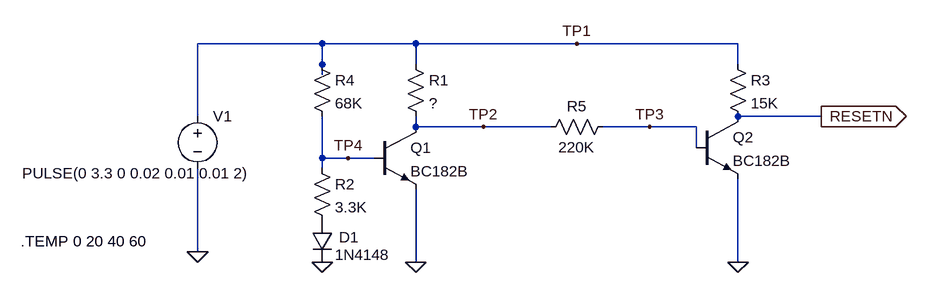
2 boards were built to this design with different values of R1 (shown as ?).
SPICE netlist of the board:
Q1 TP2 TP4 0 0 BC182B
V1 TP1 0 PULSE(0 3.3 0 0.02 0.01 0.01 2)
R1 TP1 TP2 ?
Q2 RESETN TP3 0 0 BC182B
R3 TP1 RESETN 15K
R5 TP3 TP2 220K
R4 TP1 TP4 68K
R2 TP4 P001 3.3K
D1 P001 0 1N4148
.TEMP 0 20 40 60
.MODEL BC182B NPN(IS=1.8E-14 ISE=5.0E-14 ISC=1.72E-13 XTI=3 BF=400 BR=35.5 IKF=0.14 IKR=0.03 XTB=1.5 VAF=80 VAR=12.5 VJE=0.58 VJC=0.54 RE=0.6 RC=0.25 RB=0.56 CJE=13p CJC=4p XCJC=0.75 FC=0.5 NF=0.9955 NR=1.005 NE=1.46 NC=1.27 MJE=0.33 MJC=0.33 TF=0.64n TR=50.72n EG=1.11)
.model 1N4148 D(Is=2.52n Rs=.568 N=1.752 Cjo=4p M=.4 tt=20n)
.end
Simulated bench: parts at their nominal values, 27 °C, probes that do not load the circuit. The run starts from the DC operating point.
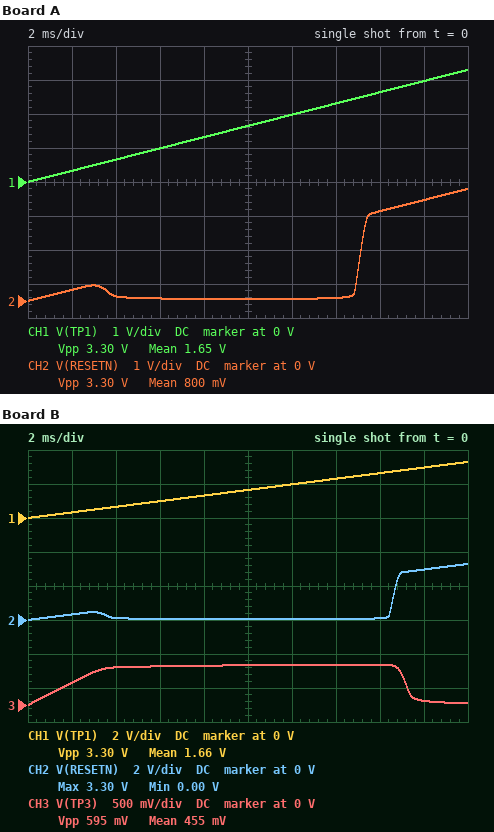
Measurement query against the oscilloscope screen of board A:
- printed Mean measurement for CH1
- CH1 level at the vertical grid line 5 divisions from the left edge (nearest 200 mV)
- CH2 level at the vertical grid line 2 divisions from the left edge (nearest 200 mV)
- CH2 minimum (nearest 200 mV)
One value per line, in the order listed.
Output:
1.65 V
1.6 V
200 mV
0 V
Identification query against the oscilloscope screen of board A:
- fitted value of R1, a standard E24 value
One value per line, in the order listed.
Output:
180 kΩ
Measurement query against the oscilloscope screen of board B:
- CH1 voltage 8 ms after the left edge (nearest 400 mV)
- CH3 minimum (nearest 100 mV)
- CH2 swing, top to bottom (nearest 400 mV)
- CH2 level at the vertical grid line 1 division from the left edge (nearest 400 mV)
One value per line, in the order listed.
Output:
1.2 V
0 V
3.2 V
400 mV
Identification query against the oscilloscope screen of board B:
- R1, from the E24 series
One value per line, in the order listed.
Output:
110 kΩ
